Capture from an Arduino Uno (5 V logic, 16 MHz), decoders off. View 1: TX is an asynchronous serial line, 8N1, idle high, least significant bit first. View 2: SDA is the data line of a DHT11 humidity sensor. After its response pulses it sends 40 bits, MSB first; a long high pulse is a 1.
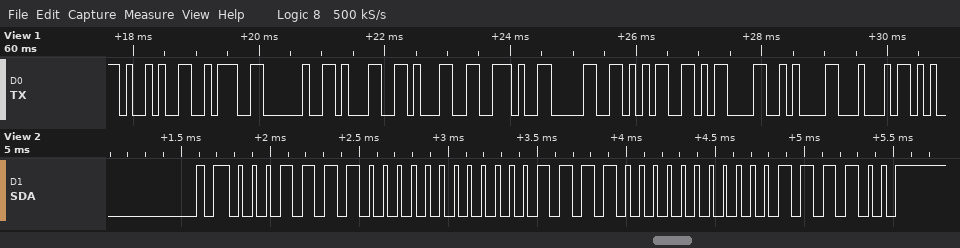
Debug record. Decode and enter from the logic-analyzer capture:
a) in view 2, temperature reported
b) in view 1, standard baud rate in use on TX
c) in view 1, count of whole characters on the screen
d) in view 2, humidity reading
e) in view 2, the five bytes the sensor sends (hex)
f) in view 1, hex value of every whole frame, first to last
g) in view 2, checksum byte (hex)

30.0 °C
9600 baud
11
30 %
1E 00 1E 00 3C
29 3A 20 31 31 2E 30 35 0D 0A 44
0x3C
